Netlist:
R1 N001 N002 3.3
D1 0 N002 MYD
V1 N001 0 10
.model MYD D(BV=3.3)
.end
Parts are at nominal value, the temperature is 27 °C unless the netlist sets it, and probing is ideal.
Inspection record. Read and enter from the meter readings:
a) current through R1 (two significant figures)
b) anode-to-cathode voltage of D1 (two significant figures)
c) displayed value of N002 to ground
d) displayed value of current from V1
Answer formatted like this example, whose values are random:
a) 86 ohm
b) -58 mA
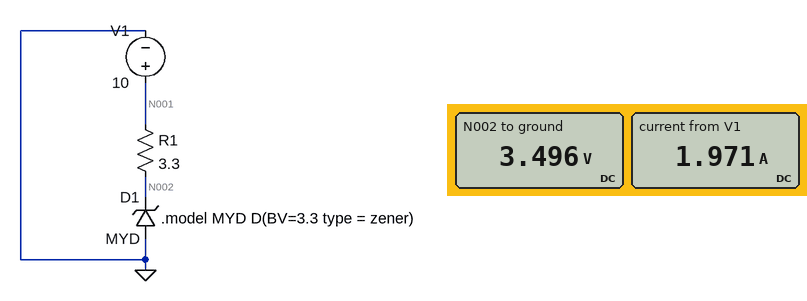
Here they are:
a) 2.0 A
b) -3.5 V
c) 3.496 V
d) 1.971 A
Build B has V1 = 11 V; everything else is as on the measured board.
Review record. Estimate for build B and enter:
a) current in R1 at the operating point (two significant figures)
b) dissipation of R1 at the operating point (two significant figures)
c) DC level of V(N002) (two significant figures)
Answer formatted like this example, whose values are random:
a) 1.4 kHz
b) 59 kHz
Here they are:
a) 2.3 A
b) 17 W
c) 3.5 V
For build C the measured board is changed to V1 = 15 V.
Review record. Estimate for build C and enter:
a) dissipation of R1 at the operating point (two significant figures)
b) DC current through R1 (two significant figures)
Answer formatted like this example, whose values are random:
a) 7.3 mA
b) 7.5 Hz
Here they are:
a) 40 W
b) 3.5 A
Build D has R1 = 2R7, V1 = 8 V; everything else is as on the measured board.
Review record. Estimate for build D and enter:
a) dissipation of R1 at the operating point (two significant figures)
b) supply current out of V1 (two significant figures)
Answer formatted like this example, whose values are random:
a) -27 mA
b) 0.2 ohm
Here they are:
a) 7.5 W
b) 1.7 A
